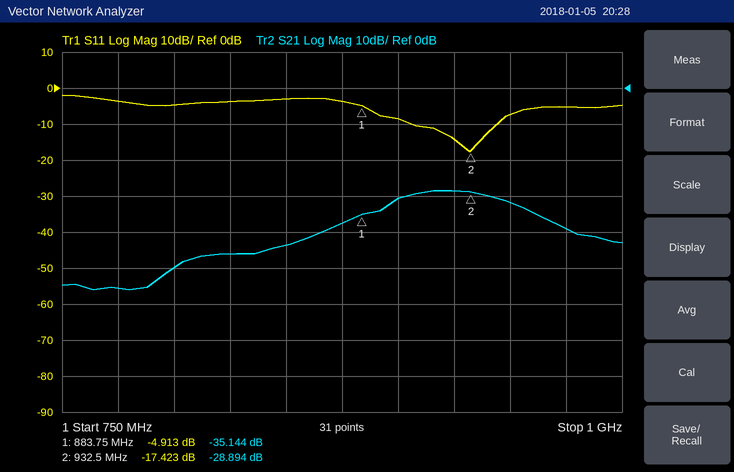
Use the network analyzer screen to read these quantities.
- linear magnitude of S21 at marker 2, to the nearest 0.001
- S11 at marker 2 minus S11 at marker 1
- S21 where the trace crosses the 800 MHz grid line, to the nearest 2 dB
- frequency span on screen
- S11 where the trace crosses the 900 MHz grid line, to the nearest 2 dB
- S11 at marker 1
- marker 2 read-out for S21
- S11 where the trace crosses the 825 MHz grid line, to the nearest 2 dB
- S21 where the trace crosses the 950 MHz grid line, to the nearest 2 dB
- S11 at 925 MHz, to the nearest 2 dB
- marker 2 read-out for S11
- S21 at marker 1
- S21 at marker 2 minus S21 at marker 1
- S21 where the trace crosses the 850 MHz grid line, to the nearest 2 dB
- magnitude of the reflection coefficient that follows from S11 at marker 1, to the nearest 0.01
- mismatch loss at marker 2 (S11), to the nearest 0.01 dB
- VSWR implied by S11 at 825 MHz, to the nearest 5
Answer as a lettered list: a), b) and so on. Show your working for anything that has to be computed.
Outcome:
a) 10^(-28.894/20) ≈ 0.036
b) -17.423 − (-4.913) = -12.510 dB
c) -50 dB
d) 250 MHz
e) -8 dB
f) -4.913 dB
g) -28.894 dB
h) -4 dB
i) -32 dB
j) -14 dB
k) -17.423 dB
l) -35.144 dB
m) -28.894 − (-35.144) = 6.250 dB
n) -44 dB
o) 10^(-4.913/20) ≈ 0.57
p) −10 log10(1 − 10^(-17.423/10)) ≈ 0.08 dB
q) |Γ| = 10^(-4/20) = 0.6310; VSWR = (1 + 0.6310)/(1 − 0.6310) ≈ 4.42, so 5 to the nearest 5
